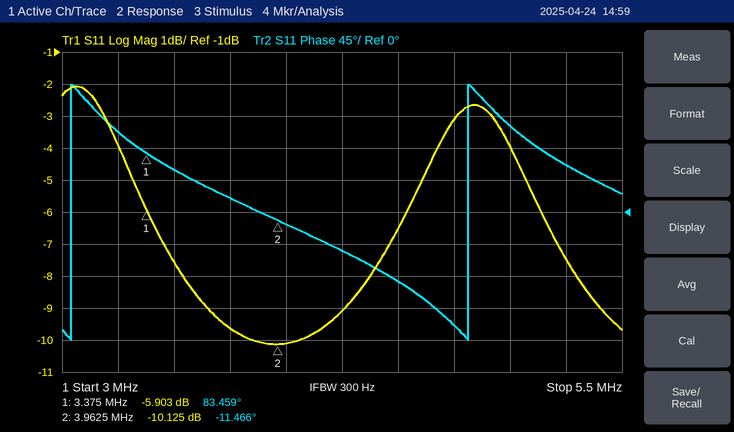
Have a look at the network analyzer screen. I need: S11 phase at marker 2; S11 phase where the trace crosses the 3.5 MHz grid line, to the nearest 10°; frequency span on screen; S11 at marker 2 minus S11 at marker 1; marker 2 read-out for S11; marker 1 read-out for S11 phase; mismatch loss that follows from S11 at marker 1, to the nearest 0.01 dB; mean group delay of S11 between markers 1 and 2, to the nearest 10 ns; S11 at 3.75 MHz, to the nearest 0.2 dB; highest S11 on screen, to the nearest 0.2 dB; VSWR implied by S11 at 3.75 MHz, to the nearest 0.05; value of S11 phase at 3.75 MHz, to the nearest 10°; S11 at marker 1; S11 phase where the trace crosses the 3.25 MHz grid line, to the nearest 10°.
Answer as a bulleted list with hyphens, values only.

- -11.466°
- 60°
- 2.5 MHz
- -4.222 dB
- -10.125 dB
- 83.459°
- 1.29 dB
- 450 ns
- -9.6 dB
- -2.0 dB
- 2.00
- 20°
- -5.903 dB
- 110°
